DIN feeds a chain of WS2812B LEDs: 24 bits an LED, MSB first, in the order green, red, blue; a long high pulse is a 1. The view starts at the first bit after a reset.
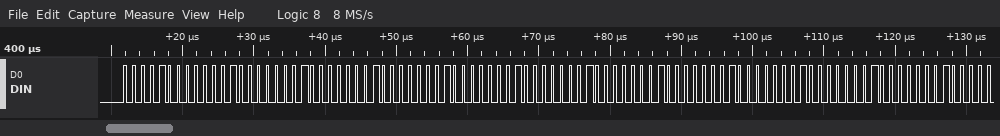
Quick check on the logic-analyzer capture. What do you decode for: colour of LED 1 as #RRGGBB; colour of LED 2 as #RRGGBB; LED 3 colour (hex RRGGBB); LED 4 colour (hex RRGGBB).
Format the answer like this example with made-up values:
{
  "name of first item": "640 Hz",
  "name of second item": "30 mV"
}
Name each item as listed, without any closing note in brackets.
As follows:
{
  "colour of LED 1 as #RRGGBB": "#080808",
  "colour of LED 2 as #RRGGBB": "#080808",
  "LED 3 colour": "#080808",
  "LED 4 colour": "#080808"
}
